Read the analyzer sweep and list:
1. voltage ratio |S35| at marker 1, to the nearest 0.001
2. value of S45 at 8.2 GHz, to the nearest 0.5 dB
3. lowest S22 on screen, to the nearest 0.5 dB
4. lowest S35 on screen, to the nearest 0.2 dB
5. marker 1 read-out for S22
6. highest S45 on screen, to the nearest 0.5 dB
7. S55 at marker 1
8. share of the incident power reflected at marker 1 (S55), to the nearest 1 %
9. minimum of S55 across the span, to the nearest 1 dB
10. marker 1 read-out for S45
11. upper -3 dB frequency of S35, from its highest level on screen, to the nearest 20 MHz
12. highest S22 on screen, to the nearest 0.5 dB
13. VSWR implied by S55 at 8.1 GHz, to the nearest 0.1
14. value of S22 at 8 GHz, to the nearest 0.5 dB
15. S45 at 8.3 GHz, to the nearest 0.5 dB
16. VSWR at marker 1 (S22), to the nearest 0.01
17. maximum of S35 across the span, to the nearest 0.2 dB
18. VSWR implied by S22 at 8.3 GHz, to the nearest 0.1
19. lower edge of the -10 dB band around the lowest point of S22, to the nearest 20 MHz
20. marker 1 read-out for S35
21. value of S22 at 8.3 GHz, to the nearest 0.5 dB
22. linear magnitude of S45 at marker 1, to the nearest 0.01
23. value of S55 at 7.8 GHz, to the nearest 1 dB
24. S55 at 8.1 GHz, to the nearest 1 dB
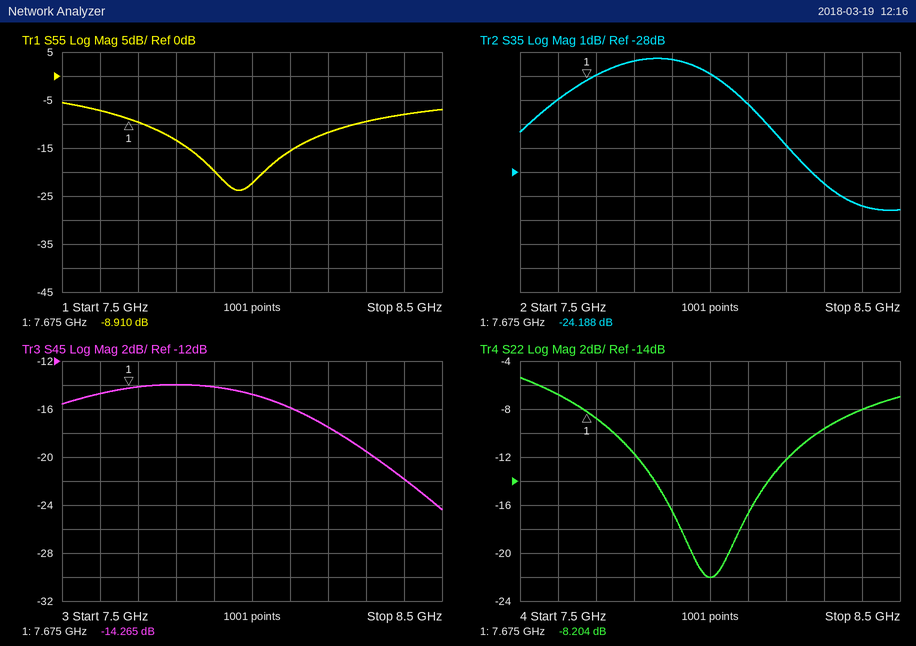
0.062
-17.5 dB
-22.0 dB
-29.6 dB
-8.204 dB
-14.0 dB
-8.910 dB
13 %
-24 dB
-14.265 dB
8.16 GHz
-5.5 dB
1.4
-22.0 dB
-19.5 dB
2.27
-23.2 dB
2.0
7.74 GHz
-24.188 dB
-9.5 dB
0.19
-13 dB
-16 dB
